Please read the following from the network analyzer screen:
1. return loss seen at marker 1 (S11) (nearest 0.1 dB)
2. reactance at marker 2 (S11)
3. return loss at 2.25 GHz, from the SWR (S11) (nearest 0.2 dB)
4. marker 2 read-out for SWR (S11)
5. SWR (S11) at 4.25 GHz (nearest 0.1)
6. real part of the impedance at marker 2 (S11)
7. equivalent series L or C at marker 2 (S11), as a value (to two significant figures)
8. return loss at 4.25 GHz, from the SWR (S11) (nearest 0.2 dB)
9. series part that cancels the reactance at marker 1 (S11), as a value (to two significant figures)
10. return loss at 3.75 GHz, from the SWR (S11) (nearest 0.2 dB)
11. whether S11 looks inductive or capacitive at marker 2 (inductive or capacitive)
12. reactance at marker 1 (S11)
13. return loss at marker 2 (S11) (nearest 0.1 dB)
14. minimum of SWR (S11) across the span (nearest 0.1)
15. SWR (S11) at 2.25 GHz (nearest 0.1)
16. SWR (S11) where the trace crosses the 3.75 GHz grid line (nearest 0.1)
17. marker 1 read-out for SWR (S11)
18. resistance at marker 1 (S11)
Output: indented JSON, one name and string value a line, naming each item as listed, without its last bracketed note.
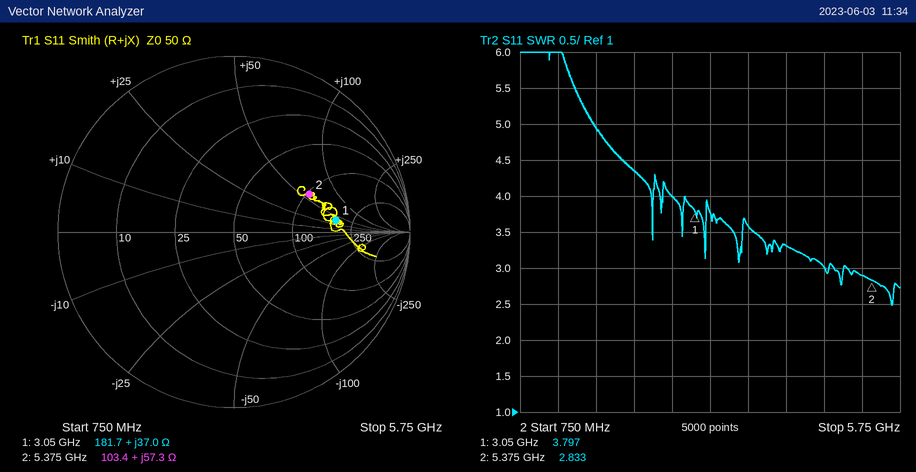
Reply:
{
  "return loss seen at marker 1 (S11)": "4.7 dB",
  "reactance at marker 2": "+57.3 Ω",
  "return loss at 2.25 GHz, from the SWR (S11)": "4.0 dB",
  "marker 2 read-out for SWR": "2.833",
  "SWR (S11) at 4.25 GHz": "3.3",
  "real part of the impedance at marker 2": "103.4 Ω",
  "equivalent series L or C at marker 2 (S11), as a value": "1.7 nH",
  "return loss at 4.25 GHz, from the SWR (S11)": "5.4 dB",
  "series part that cancels the reactance at marker 1 (S11), as a value": "1.4 pF",
  "return loss at 3.75 GHz, from the SWR (S11)": "5.0 dB",
  "whether S11 looks inductive or capacitive at marker 2": "inductive",
  "reactance at marker 1": "+37.0 Ω",
  "return loss at marker 2 (S11)": "6.4 dB",
  "minimum of SWR (S11) across the span": "2.5",
  "SWR (S11) at 2.25 GHz": "4.4",
  "SWR (S11) where the trace crosses the 3.75 GHz grid line": "3.6",
  "marker 1 read-out for SWR": "3.797",
  "resistance at marker 1": "181.7 Ω"
}
